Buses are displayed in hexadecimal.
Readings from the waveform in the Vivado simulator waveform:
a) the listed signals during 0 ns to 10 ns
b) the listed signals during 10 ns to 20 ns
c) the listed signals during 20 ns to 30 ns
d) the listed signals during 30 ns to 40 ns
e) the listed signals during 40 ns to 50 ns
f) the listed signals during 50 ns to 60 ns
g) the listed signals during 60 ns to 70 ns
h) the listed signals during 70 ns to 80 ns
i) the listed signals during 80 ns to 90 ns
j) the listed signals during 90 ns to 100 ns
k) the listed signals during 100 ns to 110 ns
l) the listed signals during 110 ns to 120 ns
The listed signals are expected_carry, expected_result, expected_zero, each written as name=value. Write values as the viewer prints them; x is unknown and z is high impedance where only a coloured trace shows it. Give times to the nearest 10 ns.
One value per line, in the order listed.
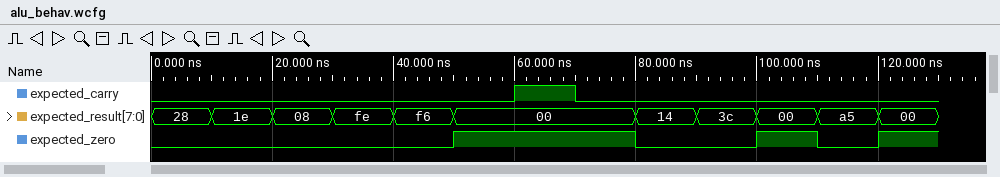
expected_carry=0, expected_result=28, expected_zero=0
expected_carry=0, expected_result=1e, expected_zero=0
expected_carry=0, expected_result=08, expected_zero=0
expected_carry=0, expected_result=fe, expected_zero=0
expected_carry=0, expected_result=f6, expected_zero=0
expected_carry=0, expected_result=00, expected_zero=1
expected_carry=1, expected_result=00, expected_zero=1
expected_carry=0, expected_result=00, expected_zero=1
expected_carry=0, expected_result=14, expected_zero=0
expected_carry=0, expected_result=3c, expected_zero=0
expected_carry=0, expected_result=00, expected_zero=1
expected_carry=0, expected_result=a5, expected_zero=0
